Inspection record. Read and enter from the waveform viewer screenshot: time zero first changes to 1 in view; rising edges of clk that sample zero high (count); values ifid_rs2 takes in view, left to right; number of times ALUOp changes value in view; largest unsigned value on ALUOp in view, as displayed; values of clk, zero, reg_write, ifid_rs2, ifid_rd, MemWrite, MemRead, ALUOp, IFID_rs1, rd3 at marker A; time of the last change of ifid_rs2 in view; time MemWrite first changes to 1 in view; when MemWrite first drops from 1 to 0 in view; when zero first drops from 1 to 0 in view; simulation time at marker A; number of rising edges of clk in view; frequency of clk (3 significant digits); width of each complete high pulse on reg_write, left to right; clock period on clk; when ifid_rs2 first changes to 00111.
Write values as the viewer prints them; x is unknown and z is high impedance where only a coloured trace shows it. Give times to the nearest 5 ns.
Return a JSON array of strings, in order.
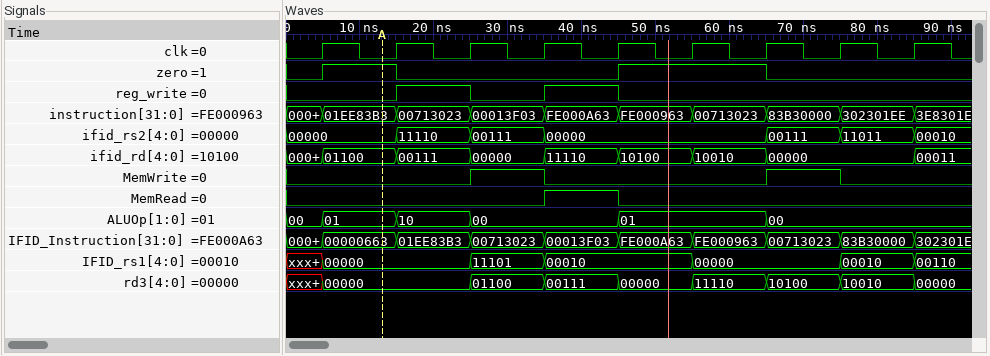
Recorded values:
["5 ns", "3", "00000, 11110, 00111, 00000, 00111, 11011, 00010", "5", "10", "clk=0, zero=1, reg_write=0, ifid_rs2=00000, ifid_rd=01100, MemWrite=0, MemRead=0, ALUOp=01, IFID_rs1=00000, rd3=00000", "85 ns", "25 ns", "35 ns", "15 ns", "15 ns", "9", "100 MHz", "10 ns, 10 ns", "10 ns", "25 ns"]
